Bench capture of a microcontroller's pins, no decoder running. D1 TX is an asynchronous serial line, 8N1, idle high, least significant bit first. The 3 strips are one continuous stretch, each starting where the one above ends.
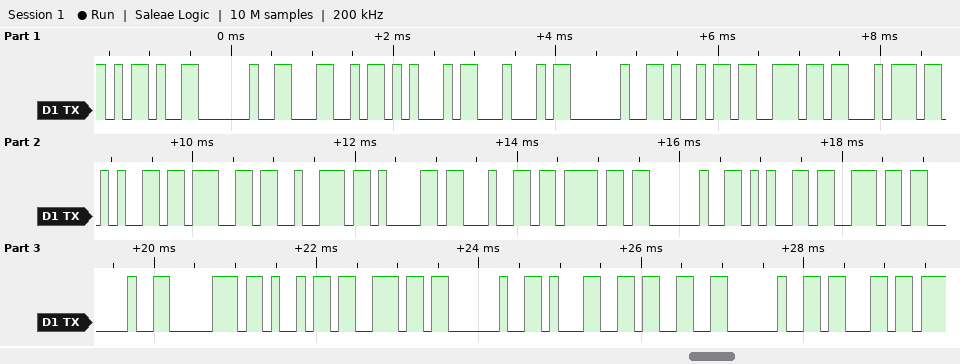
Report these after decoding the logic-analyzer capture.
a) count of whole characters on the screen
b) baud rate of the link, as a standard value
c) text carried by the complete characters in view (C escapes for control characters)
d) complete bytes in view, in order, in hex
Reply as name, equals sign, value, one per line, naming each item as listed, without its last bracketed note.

count of whole characters on the screen = 27
baud rate of the link, as a standard value = 9600 baud
text carried by the complete characters in view = "- LED integrado en pin 13 c"
complete bytes in view, in order, in hex = 2D 20 4C 45 44 20 69 6E 74 65 67 72 61 64 6F 20 65 6E 20 70 69 6E 20 31 33 20 63
